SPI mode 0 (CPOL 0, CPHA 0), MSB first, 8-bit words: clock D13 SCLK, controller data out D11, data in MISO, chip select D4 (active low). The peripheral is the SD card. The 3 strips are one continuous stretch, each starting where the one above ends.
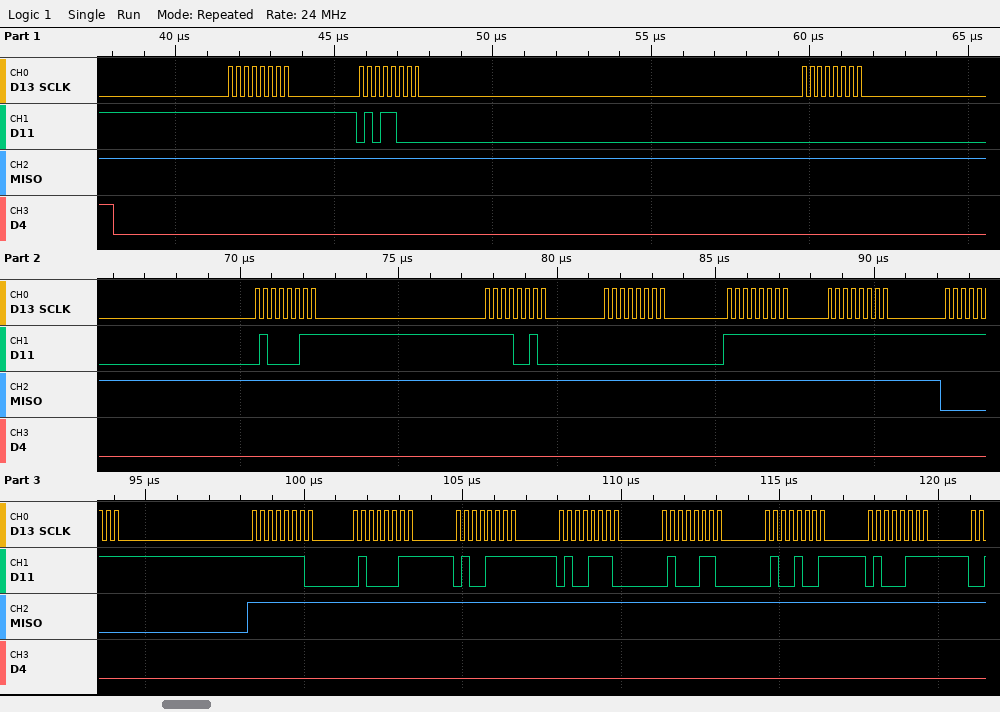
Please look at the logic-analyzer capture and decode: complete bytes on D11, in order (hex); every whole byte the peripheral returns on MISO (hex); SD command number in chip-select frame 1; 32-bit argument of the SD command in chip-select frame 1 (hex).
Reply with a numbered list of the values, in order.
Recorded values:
1. FF 58 00 43 F2 00 FF FF FF FE 43 4F 4E 46 49 47
2. FF FF FF FF FF FF FF FF 00 FF FF FF FF FF FF FF
3. CMD24
4. 0x0043F200
